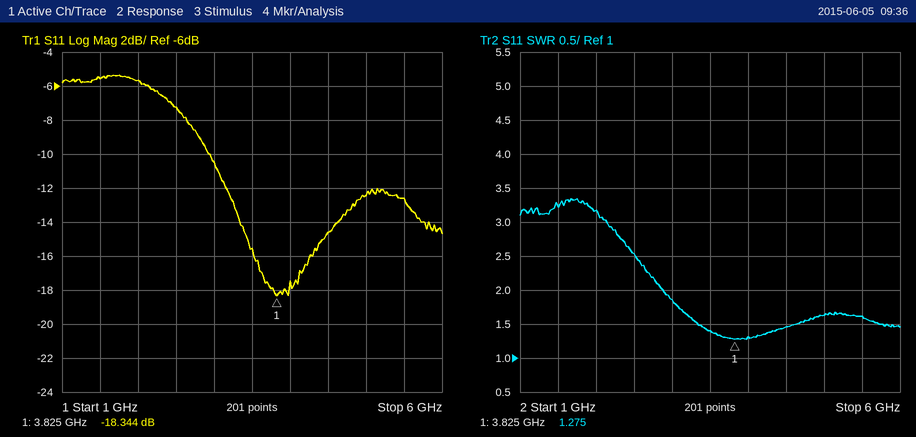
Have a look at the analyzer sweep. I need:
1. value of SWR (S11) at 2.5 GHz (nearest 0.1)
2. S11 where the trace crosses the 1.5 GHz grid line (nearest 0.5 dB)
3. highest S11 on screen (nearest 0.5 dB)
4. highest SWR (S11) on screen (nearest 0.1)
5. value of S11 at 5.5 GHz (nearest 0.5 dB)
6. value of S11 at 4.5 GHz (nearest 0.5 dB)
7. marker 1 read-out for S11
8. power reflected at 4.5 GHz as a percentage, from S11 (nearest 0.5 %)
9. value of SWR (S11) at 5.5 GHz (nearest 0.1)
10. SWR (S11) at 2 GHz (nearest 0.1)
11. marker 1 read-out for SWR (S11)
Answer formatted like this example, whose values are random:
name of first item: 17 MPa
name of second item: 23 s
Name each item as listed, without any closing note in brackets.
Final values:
value of SWR (S11) at 2.5 GHz: 2.5
S11 where the trace crosses the 1.5 GHz grid line: -5.5 dB
highest S11 on screen: -5.5 dB
highest SWR (S11) on screen: 3.3
value of S11 at 5.5 GHz: -12.5 dB
value of S11 at 4.5 GHz: -14.5 dB
marker 1 read-out for S11: -18.344 dB
power reflected at 4.5 GHz as a percentage, from S11: 3.5 %
value of SWR (S11) at 5.5 GHz: 1.6
SWR (S11) at 2 GHz: 3.2
marker 1 read-out for SWR: 1.275
